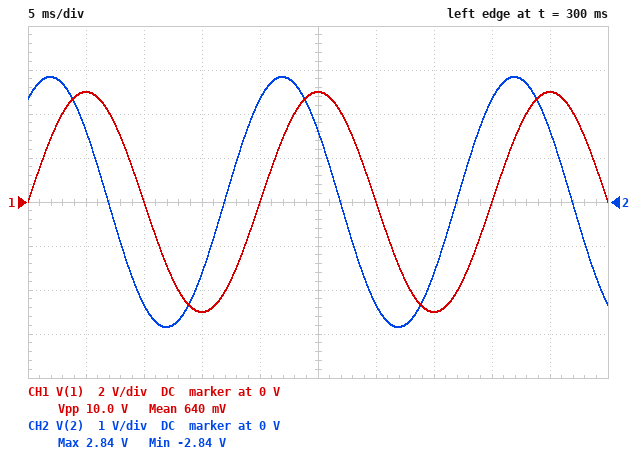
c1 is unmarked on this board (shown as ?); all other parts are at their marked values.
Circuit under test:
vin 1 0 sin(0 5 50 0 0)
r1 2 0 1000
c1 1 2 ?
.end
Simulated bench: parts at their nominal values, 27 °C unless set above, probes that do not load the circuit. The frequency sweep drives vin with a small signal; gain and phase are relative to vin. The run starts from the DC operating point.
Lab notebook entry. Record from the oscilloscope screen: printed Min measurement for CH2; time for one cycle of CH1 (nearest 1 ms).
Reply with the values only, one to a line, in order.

-2.84 V
20 ms
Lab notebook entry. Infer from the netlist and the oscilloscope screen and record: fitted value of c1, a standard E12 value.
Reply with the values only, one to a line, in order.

2.2 µF
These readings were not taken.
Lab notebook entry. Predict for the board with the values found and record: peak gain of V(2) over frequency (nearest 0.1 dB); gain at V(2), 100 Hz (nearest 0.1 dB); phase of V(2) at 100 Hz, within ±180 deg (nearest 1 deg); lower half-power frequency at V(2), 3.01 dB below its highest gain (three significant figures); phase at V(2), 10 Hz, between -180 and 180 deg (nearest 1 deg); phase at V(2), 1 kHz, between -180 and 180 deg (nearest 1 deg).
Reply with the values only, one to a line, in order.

0 dB
-1.8 dB
36 deg
72.3 Hz
82 deg
4 deg
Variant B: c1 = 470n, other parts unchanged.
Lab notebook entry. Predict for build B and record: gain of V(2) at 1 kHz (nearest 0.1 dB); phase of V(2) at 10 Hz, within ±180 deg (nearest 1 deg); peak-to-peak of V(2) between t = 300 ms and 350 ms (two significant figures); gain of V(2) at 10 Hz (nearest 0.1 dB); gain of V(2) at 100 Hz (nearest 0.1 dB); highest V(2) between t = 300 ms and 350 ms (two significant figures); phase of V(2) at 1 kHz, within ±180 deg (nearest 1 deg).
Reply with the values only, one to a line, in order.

-0.5 dB
88 deg
1.5 V
-30.6 dB
-11.0 dB
730 mV
19 deg
